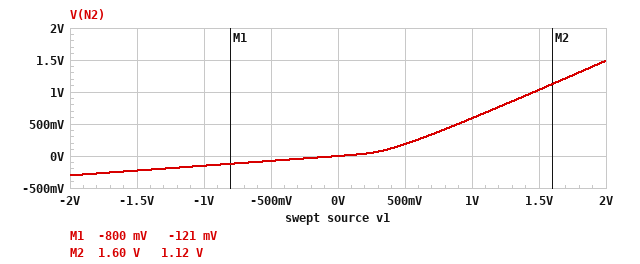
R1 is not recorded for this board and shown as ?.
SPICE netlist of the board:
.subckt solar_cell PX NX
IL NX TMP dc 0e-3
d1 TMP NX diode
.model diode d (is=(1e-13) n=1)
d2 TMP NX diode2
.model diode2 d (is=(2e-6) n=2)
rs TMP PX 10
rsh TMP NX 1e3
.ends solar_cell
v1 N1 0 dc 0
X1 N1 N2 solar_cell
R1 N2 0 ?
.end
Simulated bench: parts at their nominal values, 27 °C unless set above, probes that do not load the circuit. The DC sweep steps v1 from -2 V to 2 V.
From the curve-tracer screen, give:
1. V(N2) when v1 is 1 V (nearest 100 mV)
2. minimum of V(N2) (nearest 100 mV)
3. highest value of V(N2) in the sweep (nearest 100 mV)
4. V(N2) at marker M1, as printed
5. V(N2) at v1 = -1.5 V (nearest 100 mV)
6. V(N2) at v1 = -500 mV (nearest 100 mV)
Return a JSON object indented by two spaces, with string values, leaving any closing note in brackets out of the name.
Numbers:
{
  "V(N2) when v1 is 1 V": "600 mV",
  "minimum of V(N2)": "-300 mV",
  "highest value of V(N2) in the sweep": "1.5 V",
  "V(N2) at marker M1, as printed": "-121 mV",
  "V(N2) at v1 = -1.5 V": "-200 mV",
  "V(N2) at v1 = -500 mV": "-100 mV"
}
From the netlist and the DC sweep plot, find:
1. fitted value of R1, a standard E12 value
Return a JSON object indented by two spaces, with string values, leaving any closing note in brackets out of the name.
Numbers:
{
  "fitted value of R1, a standard E12 value": "180 Ω"
}
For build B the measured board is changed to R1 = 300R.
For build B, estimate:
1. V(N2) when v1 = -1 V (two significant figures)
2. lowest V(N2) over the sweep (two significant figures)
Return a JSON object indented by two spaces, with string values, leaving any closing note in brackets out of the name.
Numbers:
{
  "V(N2) when v1 = -1 V": "-230 mV",
  "lowest V(N2) over the sweep": "-460 mV"
}
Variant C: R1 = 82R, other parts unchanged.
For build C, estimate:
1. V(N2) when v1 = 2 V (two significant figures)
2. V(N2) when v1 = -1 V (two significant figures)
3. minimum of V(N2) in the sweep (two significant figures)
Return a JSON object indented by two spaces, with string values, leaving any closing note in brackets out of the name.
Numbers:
{
  "V(N2) when v1 = 2 V": "1.4 V",
  "V(N2) when v1 = -1 V": "-75 mV",
  "minimum of V(N2) in the sweep": "-150 mV"
}
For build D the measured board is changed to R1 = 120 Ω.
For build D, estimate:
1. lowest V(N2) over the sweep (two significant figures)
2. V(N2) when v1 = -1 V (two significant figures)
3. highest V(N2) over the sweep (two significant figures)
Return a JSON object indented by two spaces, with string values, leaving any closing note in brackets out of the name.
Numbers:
{
  "lowest V(N2) over the sweep": "-210 mV",
  "V(N2) when v1 = -1 V": "-110 mV",
  "highest V(N2) over the sweep": "1.4 V"
}
